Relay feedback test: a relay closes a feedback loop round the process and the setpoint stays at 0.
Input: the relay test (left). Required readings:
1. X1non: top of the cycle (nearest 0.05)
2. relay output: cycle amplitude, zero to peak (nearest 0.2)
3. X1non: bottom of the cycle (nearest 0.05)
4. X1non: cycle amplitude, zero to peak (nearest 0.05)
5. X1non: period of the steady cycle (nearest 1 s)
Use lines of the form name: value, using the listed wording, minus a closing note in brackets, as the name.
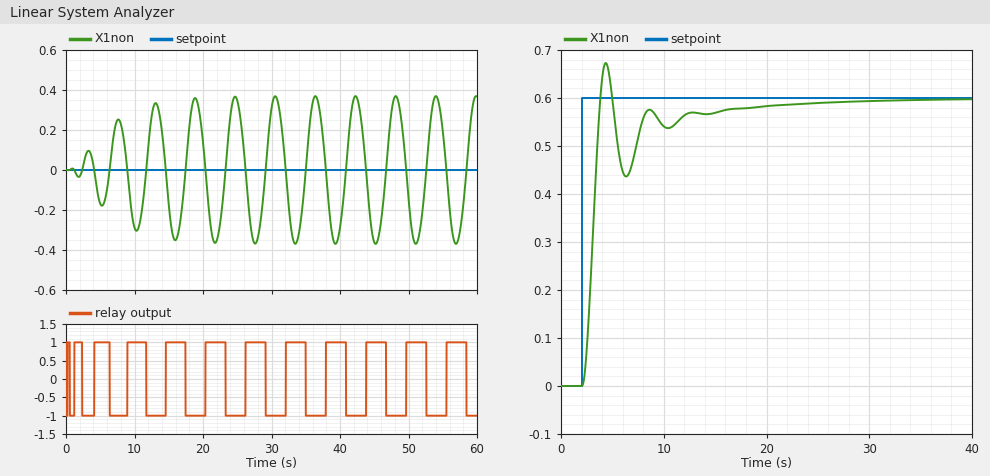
X1non: top of the cycle: 0.35
relay output: cycle amplitude, zero to peak: 1.0
X1non: bottom of the cycle: -0.35
X1non: cycle amplitude, zero to peak: 0.35
X1non: period of the steady cycle: 6 s
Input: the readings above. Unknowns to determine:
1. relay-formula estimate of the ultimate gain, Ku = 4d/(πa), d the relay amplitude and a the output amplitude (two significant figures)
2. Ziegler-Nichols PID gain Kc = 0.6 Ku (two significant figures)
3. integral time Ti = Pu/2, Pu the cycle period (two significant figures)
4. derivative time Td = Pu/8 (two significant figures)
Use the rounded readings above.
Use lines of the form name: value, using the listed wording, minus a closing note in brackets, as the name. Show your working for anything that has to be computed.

relay-formula estimate of the ultimate gain, Ku = 4d/(πa), d the relay amplitude and a the output amplitude: 4 × 1 / (π × 0.35) = 3.6
Ziegler-Nichols PID gain Kc = 0.6 Ku: 0.6 × 3.6 = 2.2
integral time Ti = Pu/2, Pu the cycle period: 6 / 2 = 3.0 s
derivative time Td = Pu/8: 6 / 8 = 0.75 s
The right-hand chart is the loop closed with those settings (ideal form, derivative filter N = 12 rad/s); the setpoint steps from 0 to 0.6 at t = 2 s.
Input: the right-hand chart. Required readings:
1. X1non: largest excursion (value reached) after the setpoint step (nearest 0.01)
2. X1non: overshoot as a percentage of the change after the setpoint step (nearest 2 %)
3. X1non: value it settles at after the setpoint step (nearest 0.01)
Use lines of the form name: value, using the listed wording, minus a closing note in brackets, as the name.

X1non: largest excursion (value reached) after the setpoint step: 0.67
X1non: overshoot as a percentage of the change after the setpoint step: 12 %
X1non: value it settles at after the setpoint step: 0.60
